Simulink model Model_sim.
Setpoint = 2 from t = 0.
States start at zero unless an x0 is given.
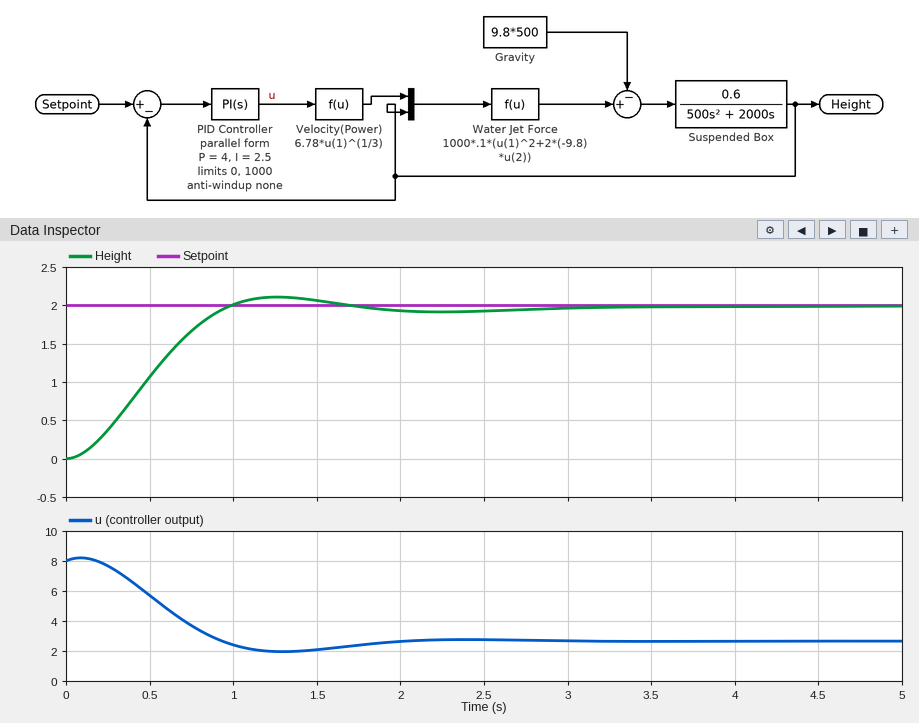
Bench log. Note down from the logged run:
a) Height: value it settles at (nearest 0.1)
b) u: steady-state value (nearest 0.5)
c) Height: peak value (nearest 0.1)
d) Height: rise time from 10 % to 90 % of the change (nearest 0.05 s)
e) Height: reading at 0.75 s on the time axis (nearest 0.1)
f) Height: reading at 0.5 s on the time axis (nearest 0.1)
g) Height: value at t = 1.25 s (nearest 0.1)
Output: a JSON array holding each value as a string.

["2.0", "2.5", "2.1", "0.65 s", "1.7", "1.1", "2.1"]
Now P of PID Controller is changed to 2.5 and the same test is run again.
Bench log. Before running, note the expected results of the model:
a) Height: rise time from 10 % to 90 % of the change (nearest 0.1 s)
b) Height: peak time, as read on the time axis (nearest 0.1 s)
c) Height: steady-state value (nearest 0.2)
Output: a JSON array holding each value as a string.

["0.8 s", "1.8 s", "2.0"]
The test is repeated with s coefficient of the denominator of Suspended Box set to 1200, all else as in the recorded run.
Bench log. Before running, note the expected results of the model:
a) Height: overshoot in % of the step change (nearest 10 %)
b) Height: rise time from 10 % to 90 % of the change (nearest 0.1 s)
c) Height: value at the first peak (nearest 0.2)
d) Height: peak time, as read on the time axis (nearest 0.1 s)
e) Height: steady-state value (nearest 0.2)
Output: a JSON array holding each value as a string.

["20 %", "0.5 s", "2.4", "1.0 s", "2.0"]
